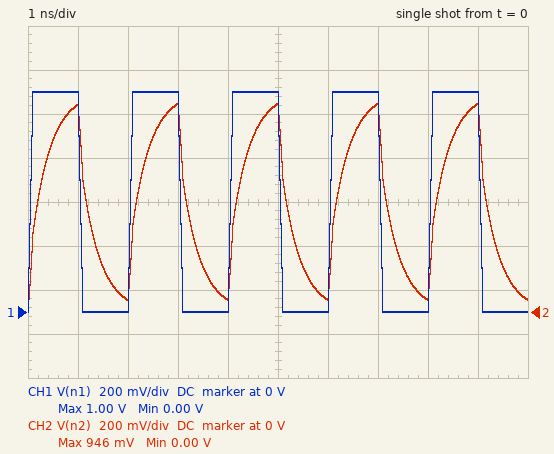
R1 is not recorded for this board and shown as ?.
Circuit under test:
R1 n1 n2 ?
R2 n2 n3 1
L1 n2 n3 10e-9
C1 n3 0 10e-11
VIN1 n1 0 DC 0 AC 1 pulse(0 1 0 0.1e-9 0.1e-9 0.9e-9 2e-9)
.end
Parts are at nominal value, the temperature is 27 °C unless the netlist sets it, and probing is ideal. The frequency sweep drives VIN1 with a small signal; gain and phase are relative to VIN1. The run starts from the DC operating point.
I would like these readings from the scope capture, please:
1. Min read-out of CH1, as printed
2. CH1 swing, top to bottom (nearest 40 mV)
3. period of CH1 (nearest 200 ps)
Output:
0.00 V
1.00 V
2.0 ns
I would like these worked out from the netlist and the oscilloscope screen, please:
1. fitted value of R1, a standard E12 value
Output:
2.7 Ω
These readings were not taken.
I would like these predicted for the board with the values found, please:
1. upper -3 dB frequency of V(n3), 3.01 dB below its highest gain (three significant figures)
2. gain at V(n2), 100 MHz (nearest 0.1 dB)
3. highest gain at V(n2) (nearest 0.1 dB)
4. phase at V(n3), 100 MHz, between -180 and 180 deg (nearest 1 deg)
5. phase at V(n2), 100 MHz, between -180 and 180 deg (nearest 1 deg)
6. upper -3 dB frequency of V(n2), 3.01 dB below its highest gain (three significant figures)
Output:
430 MHz
-0.2 dB
0 dB
-13 deg
-10 deg
461 MHz
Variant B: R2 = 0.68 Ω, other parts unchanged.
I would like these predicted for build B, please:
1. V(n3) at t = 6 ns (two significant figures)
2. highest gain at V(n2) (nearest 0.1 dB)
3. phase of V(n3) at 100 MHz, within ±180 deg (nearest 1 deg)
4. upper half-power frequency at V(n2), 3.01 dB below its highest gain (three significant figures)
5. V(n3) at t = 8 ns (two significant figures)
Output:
58 mV
0 dB
-12 deg
489 MHz
57 mV
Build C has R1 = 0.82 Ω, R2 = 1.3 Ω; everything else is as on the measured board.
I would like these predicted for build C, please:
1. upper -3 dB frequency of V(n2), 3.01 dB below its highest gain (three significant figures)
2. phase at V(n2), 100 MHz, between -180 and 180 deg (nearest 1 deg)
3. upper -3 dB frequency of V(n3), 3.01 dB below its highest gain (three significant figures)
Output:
1.48 GHz
-3 deg
745 MHz
